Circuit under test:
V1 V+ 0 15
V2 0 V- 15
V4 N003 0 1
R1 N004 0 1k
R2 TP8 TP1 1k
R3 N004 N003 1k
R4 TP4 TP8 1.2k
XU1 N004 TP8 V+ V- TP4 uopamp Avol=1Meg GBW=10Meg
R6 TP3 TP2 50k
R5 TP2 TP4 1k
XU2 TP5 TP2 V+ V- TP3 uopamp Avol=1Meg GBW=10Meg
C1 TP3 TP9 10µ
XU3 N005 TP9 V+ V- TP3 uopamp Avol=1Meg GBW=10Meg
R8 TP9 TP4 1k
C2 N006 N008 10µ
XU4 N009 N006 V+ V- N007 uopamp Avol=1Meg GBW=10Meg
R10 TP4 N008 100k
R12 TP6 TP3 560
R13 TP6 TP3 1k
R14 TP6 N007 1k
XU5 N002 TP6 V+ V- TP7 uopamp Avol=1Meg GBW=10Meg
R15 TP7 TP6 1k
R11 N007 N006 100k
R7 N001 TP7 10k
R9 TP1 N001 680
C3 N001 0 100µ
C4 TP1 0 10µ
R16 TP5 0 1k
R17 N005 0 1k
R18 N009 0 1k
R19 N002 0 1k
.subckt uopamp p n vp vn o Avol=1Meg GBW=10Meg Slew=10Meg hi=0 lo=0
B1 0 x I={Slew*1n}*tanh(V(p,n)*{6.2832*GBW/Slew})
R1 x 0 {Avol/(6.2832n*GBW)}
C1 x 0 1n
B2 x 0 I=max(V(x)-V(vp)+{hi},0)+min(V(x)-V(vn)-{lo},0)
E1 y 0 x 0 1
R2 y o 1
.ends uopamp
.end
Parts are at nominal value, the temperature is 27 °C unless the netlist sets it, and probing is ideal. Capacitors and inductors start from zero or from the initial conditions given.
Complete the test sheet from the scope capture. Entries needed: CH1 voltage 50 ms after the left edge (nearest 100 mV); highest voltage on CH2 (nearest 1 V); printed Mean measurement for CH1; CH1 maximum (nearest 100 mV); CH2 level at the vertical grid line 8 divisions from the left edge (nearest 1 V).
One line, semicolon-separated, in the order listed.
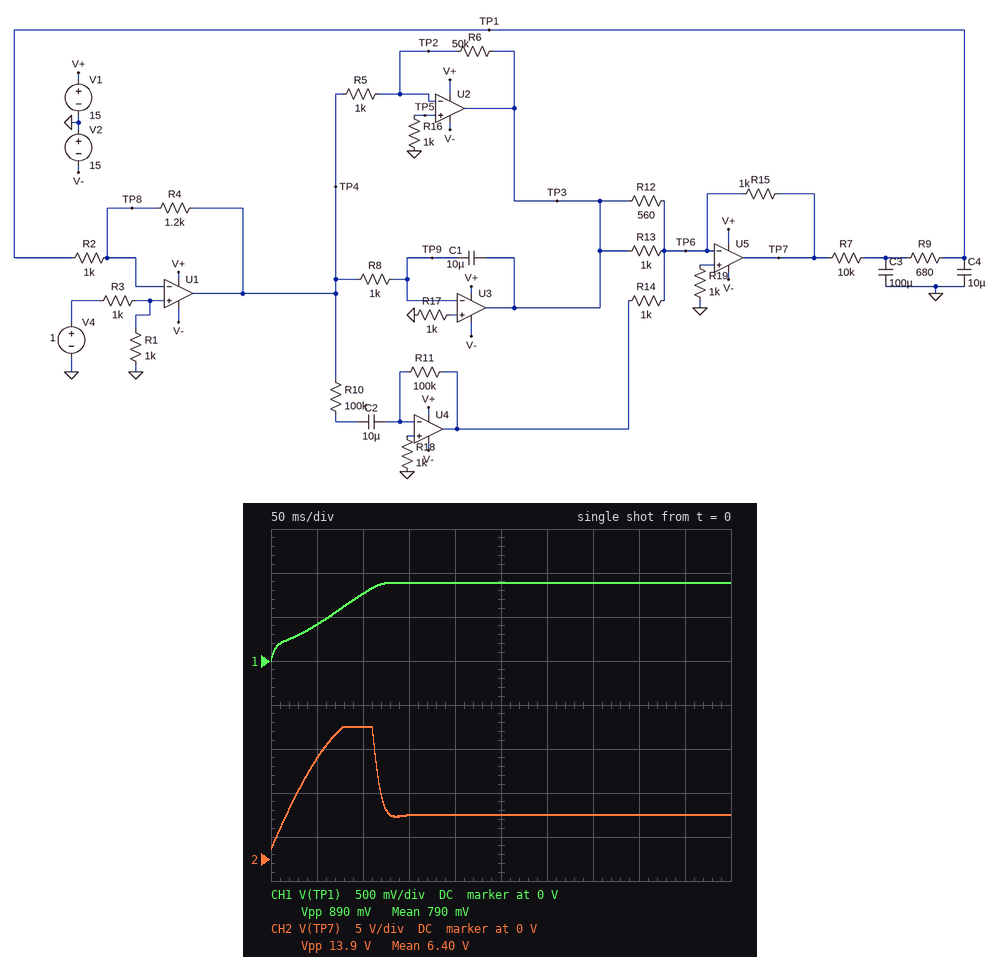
400 mV; 15 V; 790 mV; 900 mV; 5 V
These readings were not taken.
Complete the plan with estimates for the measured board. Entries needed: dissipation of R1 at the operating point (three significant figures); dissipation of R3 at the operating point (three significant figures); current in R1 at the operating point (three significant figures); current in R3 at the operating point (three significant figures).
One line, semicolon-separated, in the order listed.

250 µW; 250 µW; 500 µA; 500 µA
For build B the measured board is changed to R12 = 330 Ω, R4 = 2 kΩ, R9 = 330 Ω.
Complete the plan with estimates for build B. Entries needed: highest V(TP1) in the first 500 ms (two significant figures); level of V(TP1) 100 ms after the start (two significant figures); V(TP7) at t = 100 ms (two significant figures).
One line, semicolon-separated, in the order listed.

750 mV; 740 mV; 3.2 V
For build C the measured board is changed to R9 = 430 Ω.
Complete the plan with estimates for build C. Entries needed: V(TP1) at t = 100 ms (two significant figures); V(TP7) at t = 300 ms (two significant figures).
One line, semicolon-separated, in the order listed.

820 mV; 4.9 V
